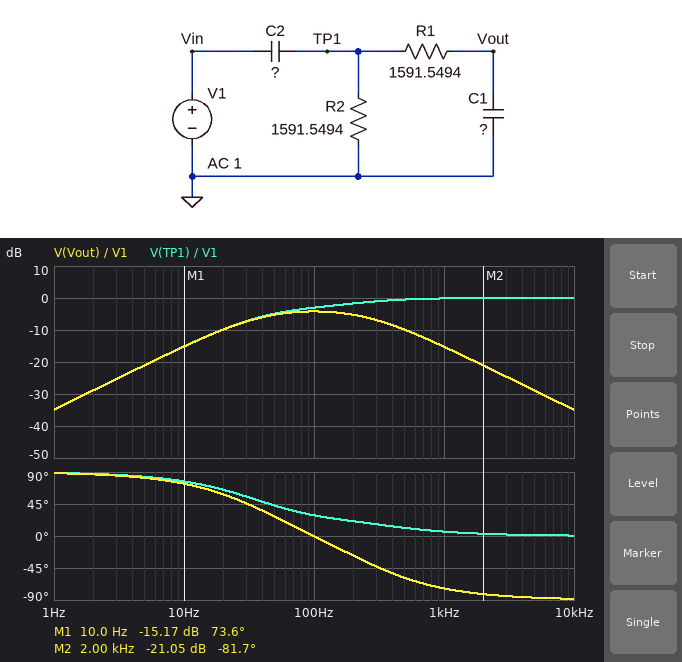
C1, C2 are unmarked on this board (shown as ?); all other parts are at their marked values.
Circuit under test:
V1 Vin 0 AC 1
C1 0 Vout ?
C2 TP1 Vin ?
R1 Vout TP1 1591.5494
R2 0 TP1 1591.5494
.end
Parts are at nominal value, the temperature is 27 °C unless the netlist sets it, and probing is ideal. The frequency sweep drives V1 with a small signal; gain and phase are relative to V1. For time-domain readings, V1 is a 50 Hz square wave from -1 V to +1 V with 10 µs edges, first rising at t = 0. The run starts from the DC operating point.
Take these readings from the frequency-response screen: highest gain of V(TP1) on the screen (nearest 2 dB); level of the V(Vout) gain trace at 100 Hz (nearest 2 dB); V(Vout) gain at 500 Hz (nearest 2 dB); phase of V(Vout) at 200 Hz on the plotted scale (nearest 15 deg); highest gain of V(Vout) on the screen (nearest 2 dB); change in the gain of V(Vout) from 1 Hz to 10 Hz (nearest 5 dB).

0 dB
-4 dB
-10 dB
-30 deg
-4 dB
20 dB
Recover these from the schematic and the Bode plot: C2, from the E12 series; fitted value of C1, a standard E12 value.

1.8 µF
560 nF
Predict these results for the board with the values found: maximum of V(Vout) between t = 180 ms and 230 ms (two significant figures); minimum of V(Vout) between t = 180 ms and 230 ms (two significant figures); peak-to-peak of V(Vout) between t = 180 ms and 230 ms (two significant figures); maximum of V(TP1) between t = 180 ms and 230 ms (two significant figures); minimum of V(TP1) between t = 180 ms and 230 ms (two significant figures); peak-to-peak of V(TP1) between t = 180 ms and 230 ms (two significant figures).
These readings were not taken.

920 mV
-920 mV
1.8 V
1.9 V
-1.9 V
3.8 V
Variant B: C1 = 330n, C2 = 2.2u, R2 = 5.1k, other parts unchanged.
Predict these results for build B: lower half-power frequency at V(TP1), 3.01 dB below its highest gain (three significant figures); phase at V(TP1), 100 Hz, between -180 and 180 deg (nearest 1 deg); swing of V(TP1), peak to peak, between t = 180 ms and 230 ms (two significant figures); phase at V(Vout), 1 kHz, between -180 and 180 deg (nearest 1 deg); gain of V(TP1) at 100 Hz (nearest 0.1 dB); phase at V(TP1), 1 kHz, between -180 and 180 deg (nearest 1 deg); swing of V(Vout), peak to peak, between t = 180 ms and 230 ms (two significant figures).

17.4 Hz
9 deg
2.9 V
-70 deg
-1.2 dB
3 deg
2.1 V
